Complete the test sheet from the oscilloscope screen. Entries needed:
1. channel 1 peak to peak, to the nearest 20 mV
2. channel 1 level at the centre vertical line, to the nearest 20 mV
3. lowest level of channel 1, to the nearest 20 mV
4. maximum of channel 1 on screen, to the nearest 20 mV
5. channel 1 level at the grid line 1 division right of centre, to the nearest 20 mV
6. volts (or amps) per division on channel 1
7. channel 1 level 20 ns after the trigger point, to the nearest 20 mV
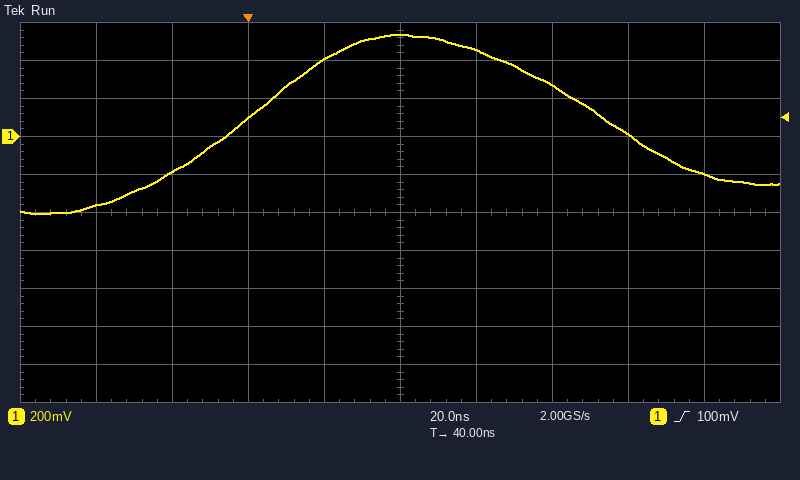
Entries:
940 mV
540 mV
-400 mV
540 mV
460 mV
200 mV
400 mV
